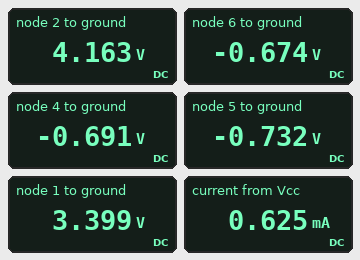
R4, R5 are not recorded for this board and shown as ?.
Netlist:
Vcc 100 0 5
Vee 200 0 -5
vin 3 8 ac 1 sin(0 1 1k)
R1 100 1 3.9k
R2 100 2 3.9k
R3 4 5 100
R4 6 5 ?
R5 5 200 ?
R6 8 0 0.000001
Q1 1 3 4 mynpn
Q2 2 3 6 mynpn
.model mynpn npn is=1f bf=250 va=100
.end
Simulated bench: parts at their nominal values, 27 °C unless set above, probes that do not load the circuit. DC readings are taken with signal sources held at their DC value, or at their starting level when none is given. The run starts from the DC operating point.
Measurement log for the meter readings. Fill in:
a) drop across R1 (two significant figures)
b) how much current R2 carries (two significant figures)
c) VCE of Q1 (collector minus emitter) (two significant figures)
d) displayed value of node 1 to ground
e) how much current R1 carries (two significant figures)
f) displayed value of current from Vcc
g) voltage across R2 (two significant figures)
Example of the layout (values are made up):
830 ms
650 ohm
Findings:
1.6 V
210 µA
4.1 V
3.399 V
410 µA
0.625 mA
840 mV
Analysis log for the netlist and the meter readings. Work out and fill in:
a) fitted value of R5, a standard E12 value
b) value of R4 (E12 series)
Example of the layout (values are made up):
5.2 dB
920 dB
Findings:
6.8 kΩ
270 Ω
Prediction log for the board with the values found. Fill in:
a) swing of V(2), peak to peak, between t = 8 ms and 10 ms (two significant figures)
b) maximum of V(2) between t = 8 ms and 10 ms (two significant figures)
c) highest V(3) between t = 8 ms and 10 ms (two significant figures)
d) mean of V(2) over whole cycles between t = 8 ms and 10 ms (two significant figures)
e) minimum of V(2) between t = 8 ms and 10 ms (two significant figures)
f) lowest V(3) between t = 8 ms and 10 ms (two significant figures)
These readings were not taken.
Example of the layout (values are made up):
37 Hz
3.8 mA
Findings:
330 mV
4.3 V
1.0 V
4.2 V
4.0 V
-1.0 V
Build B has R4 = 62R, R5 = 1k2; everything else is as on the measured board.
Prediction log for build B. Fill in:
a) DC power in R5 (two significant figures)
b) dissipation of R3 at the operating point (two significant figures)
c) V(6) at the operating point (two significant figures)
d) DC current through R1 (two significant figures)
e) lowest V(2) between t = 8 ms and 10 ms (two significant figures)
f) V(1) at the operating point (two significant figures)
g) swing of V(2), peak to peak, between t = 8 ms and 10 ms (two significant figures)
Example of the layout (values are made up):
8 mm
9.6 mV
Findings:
14 mW
200 µW
-740 mV
1.4 mA
-1.4 V
-500 mV
1.7 V
